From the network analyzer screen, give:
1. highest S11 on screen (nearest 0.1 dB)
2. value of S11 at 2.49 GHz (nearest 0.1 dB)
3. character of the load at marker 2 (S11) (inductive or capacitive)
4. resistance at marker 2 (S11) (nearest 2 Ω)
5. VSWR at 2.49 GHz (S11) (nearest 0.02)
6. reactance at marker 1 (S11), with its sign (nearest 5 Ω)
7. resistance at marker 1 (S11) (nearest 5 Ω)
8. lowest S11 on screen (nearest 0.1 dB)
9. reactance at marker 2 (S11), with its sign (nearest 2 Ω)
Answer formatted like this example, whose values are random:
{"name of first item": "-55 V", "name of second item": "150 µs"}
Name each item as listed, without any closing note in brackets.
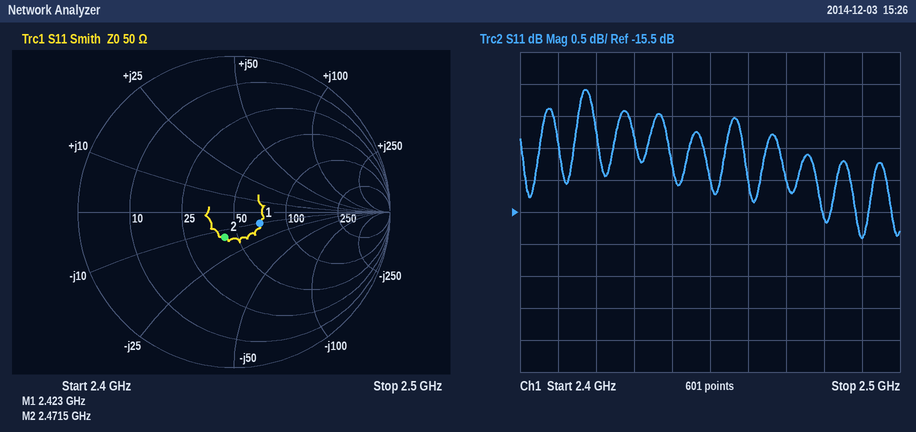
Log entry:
{"highest S11 on screen": "-13.6 dB", "value of S11 at 2.49 GHz": "-15.9 dB", "character of the load at marker 2 (S11)": "capacitive", "resistance at marker 2 (S11)": "42 Ω", "VSWR at 2.49 GHz (S11)": "1.38", "reactance at marker 1 (S11), with its sign": "-10 Ω", "resistance at marker 1 (S11)": "70 Ω", "lowest S11 on screen": "-15.9 dB", "reactance at marker 2 (S11), with its sign": "-14 Ω"}
